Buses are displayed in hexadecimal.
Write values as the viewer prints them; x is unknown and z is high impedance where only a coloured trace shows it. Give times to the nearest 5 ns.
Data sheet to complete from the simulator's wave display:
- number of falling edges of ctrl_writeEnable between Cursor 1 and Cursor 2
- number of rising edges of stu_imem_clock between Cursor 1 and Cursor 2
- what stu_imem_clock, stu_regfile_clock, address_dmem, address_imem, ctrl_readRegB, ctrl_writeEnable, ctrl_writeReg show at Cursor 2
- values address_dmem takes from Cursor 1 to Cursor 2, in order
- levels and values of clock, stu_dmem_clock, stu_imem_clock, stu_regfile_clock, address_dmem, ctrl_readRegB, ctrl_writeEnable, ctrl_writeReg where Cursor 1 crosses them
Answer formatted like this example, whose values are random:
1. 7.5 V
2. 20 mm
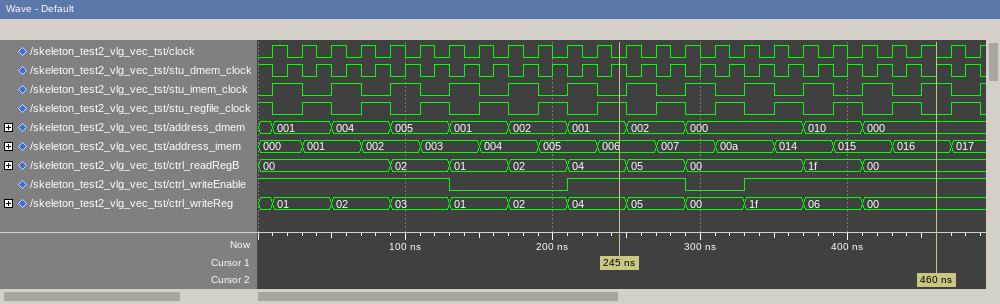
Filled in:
1. 1
2. 6
3. stu_imem_clock=1, stu_regfile_clock=0, address_dmem=000, address_imem=016, ctrl_readRegB=00, ctrl_writeEnable=1, ctrl_writeReg=00
4. 001, 002, 000, 010, 000
5. clock=0, stu_dmem_clock=1, stu_imem_clock=0, stu_regfile_clock=1, address_dmem=001, ctrl_readRegB=04, ctrl_writeEnable=1, ctrl_writeReg=04
